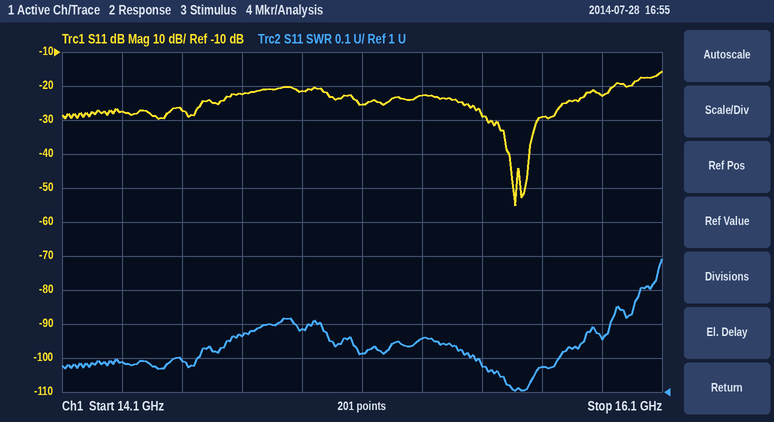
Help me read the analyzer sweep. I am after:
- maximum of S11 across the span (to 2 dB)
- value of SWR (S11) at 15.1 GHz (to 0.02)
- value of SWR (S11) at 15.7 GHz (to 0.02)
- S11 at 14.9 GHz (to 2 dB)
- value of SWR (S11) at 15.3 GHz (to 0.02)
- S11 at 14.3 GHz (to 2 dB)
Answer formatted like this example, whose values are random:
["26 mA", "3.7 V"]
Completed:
["-16 dB", "1.12", "1.08", "-22 dB", "1.16", "-28 dB"]
